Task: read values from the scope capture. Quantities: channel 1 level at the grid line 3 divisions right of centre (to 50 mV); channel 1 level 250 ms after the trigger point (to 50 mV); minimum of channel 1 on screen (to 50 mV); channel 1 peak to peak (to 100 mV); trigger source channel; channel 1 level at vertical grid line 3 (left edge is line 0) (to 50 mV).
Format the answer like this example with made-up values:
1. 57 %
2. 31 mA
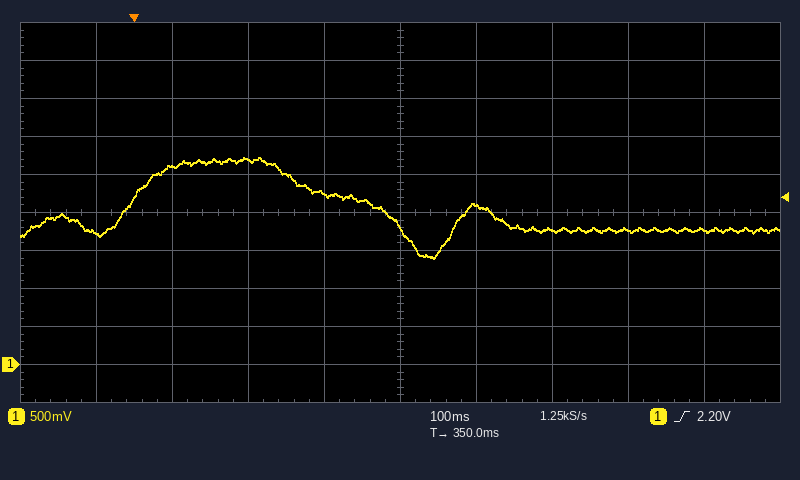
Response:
1. 1.75 V
2. 2.25 V
3. 1.40 V
4. 1.30 V
5. channel 1
6. 2.70 V
